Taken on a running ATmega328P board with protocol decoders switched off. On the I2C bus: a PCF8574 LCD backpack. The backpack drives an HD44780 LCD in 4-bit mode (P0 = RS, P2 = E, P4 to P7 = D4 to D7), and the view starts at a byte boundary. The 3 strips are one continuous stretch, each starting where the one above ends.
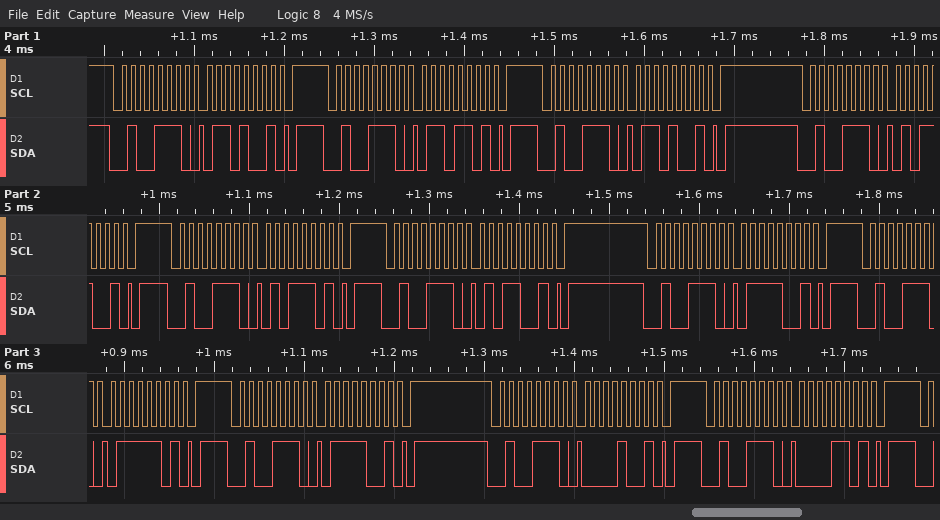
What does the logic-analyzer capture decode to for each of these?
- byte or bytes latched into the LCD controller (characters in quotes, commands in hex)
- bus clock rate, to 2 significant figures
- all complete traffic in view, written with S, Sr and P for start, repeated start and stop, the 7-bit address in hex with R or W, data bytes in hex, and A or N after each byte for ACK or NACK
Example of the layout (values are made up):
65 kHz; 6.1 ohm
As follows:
'e'; 100 kHz; S 27W A 69 A P S 27W A 6D A P S 27W A 69 A P S 27W A 59 A P S 27W A 5D A P S 27W A 59 A P S 27W A 79 A P S 27W A 7D A P S 27W A 79 A P S 27W A 09 A P S 27W A 0D A P
